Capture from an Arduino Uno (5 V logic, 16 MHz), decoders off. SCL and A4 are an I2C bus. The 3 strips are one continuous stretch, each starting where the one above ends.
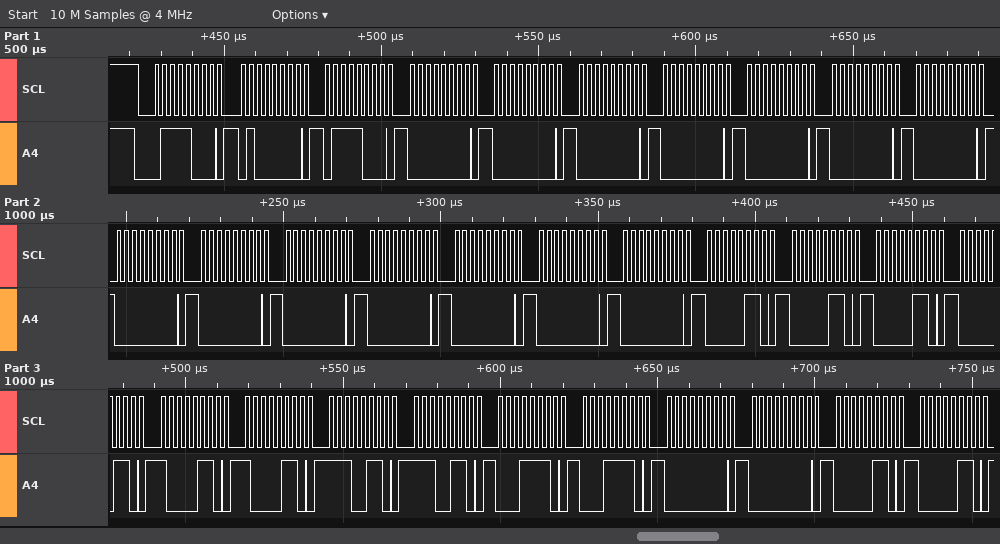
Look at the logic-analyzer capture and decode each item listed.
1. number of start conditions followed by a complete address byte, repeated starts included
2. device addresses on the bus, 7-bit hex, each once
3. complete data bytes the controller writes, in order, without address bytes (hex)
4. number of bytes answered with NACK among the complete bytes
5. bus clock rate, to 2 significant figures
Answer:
1
0x3C
40 78 00 00 00 00 00 00 00 00 00 00 00 00 00 00 06 06 06 06 86 86 E6 E6 1E 1E 00 00 06 06
0
400 kHz
